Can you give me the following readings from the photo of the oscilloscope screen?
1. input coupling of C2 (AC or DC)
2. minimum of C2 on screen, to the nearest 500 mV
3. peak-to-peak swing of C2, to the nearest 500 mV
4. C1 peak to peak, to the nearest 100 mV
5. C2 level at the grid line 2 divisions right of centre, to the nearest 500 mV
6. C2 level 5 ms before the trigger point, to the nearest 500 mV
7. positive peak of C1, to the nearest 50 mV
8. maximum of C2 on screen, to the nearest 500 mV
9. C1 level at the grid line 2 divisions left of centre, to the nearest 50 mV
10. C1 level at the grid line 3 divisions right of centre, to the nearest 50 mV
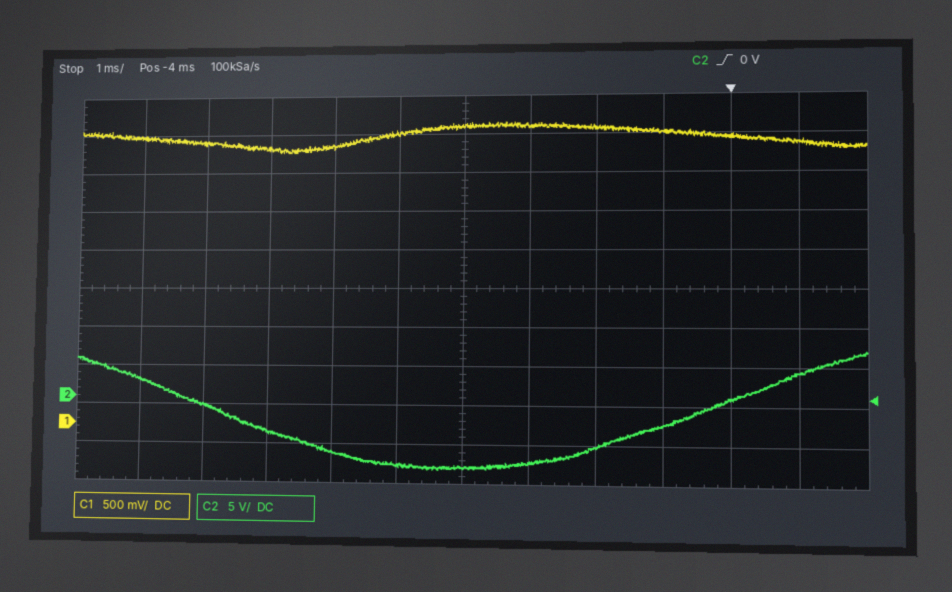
DC
-9.0 V
15.0 V
400 mV
-6.0 V
-8.5 V
3.90 V
6.0 V
3.60 V
3.75 V
